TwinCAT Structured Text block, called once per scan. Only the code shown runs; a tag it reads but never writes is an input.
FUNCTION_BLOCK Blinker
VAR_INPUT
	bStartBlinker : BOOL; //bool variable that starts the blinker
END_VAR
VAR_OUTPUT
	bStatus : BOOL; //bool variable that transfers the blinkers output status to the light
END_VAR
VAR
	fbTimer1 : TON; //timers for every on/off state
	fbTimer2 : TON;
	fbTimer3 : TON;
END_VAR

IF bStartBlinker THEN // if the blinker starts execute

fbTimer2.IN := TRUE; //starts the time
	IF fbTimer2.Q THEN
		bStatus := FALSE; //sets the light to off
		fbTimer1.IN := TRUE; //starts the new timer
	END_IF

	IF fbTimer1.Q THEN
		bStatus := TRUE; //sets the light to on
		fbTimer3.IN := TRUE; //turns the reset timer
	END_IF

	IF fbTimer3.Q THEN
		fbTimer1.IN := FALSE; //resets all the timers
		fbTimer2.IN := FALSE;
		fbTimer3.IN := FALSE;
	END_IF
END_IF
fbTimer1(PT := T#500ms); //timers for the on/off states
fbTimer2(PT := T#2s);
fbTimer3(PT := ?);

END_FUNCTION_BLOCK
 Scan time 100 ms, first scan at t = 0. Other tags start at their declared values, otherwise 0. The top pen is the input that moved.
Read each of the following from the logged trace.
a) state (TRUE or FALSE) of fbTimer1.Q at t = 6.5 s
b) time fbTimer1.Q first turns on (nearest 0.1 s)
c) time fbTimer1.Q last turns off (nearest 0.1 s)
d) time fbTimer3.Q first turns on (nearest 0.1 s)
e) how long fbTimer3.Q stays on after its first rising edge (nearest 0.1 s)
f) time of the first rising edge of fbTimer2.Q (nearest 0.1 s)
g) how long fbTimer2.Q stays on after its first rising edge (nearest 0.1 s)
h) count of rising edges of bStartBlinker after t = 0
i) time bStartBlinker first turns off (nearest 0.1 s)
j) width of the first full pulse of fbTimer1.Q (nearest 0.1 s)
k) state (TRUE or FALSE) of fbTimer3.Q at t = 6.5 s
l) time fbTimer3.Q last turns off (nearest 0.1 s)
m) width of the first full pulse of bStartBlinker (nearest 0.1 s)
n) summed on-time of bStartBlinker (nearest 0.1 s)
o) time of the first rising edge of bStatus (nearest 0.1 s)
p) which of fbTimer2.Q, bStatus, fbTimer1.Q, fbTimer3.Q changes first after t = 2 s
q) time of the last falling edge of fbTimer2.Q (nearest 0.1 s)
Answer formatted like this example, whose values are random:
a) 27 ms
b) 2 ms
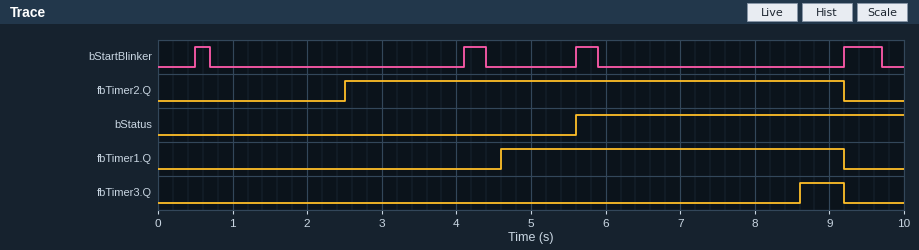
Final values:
a) TRUE
b) 4.6 s
c) 9.2 s
d) 8.6 s
e) 0.6 s
f) 2.5 s
g) 6.7 s
h) 4
i) 0.7 s
j) 4.6 s
k) FALSE
l) 9.2 s
m) 0.2 s
n) 1.3 s
o) 5.6 s
p) fbTimer2.Q
q) 9.2 s
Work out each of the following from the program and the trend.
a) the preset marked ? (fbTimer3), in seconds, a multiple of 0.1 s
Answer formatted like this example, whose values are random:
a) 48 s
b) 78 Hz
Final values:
a) 3.0 s
